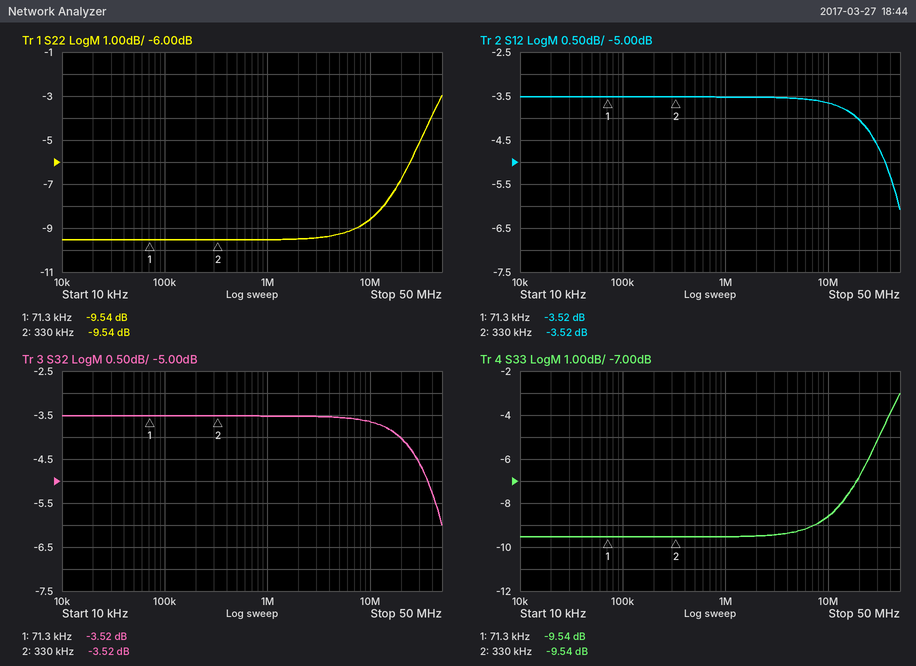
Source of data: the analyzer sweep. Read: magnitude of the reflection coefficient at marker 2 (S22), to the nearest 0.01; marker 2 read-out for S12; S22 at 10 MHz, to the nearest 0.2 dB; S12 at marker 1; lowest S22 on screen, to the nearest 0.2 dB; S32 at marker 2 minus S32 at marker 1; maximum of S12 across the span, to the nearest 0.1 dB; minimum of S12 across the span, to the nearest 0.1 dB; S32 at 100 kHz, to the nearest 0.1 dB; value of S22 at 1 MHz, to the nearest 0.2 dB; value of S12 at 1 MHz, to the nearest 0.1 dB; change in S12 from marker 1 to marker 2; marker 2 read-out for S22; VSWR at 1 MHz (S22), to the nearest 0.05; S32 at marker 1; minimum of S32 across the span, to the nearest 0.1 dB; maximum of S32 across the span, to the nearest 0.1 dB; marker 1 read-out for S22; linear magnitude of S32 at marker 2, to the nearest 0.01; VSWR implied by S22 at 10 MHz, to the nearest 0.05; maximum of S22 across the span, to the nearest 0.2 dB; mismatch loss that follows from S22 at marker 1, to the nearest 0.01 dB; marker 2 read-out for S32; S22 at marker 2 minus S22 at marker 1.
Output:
0.33
-3.52 dB
-8.6 dB
-3.52 dB
-9.6 dB
0.00 dB
-3.5 dB
-6.1 dB
-3.5 dB
-9.6 dB
-3.5 dB
0.00 dB
-9.54 dB
2.00
-3.52 dB
-6.0 dB
-3.5 dB
-9.54 dB
0.67
2.20
-3.0 dB
0.51 dB
-3.52 dB
0.00 dB
